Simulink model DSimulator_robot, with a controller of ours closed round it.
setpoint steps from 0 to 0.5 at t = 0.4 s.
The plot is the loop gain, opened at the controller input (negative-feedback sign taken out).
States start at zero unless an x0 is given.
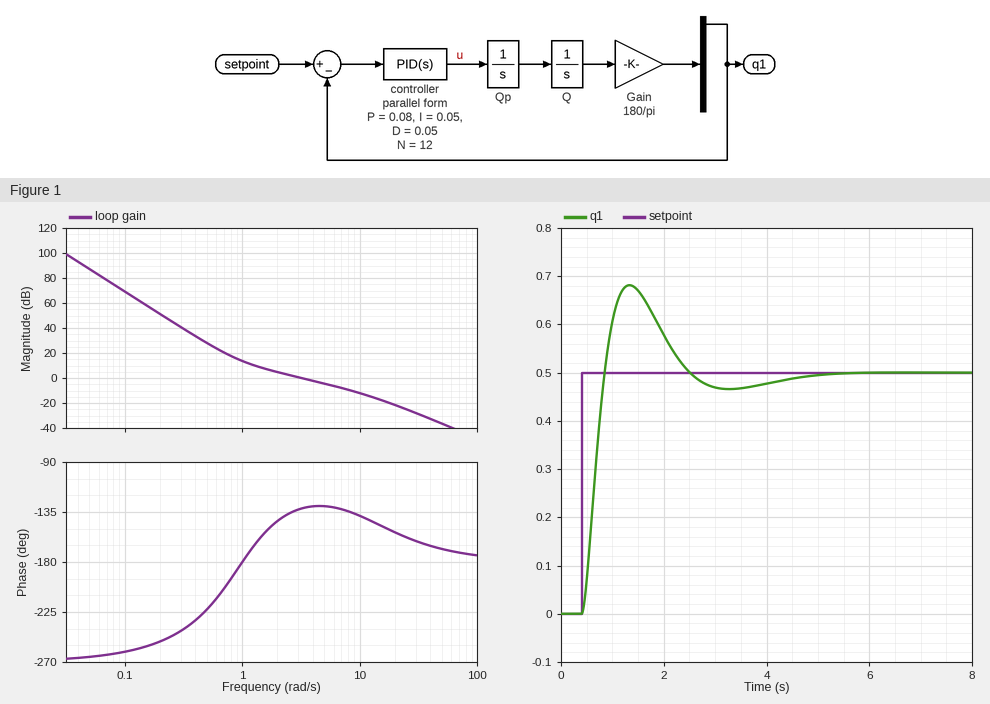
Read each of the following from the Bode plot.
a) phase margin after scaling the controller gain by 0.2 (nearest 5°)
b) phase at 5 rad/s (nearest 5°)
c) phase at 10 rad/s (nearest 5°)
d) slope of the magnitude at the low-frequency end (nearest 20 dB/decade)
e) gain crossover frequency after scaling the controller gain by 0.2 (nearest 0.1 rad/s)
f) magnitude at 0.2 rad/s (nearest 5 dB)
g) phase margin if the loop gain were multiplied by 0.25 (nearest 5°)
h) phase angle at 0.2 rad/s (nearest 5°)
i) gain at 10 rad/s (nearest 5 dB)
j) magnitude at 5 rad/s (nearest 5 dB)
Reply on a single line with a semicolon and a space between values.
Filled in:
0°; -130°; -140°; -60 dB/decade; 1.0 rad/s; 50 dB; 5°; -250°; -10 dB; -5 dB
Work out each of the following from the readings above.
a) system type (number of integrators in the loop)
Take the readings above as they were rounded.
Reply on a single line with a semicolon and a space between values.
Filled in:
3
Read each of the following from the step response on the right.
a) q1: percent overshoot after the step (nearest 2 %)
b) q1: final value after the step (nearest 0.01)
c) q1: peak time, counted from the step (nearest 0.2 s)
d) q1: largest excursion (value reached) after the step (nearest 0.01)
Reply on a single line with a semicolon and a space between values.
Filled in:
36 %; 0.50; 1.0 s; 0.68
